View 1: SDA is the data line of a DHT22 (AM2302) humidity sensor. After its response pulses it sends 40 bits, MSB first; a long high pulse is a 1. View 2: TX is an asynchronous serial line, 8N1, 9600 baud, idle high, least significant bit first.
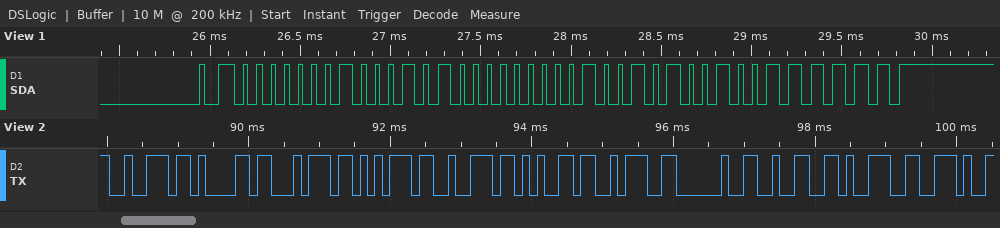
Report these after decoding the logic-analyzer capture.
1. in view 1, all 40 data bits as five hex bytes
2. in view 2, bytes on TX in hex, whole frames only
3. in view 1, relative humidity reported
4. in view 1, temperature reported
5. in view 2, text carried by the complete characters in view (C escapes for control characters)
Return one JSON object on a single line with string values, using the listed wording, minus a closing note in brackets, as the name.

{"in view 1, all 40 data bits as five hex bytes": "01 14 01 29 3F", "in view 2, bytes on TX in hex, whole frames only": "72 61 74 75 72 65 3A 20 32 39 2E", "in view 1, relative humidity reported": "27.6 %", "in view 1, temperature reported": "29.7 °C", "in view 2, text carried by the complete characters in view": "\"rature: 29.\""}
